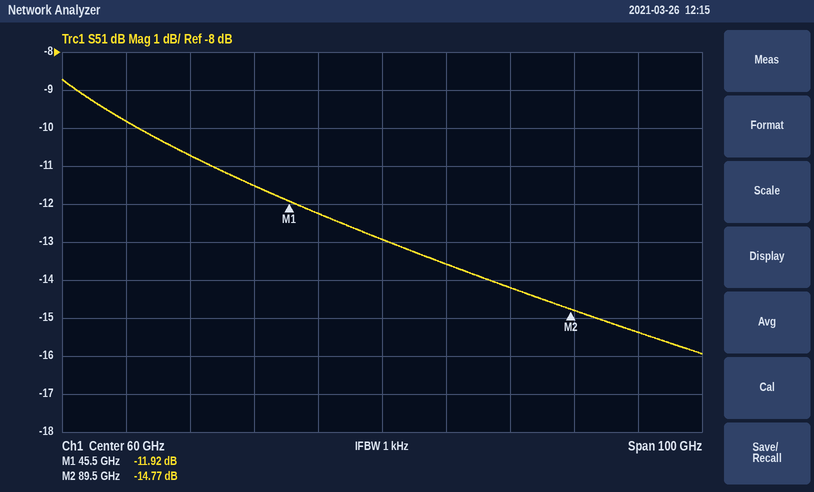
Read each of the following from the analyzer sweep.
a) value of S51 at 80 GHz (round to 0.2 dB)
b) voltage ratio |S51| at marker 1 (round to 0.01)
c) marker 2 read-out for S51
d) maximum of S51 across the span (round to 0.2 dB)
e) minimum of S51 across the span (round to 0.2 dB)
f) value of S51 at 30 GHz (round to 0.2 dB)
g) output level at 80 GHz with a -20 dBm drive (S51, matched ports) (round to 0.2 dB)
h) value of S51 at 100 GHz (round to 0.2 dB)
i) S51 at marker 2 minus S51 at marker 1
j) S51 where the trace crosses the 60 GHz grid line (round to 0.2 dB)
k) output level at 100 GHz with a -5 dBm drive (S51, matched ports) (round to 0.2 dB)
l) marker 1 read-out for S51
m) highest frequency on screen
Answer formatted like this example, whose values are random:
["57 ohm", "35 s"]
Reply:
["-14.2 dB", "0.25", "-14.77 dB", "-8.8 dB", "-16.0 dB", "-10.8 dB", "-34.2 dBm", "-15.4 dB", "-2.85 dB", "-13.0 dB", "-20.4 dBm", "-11.92 dB", "110 GHz"]
